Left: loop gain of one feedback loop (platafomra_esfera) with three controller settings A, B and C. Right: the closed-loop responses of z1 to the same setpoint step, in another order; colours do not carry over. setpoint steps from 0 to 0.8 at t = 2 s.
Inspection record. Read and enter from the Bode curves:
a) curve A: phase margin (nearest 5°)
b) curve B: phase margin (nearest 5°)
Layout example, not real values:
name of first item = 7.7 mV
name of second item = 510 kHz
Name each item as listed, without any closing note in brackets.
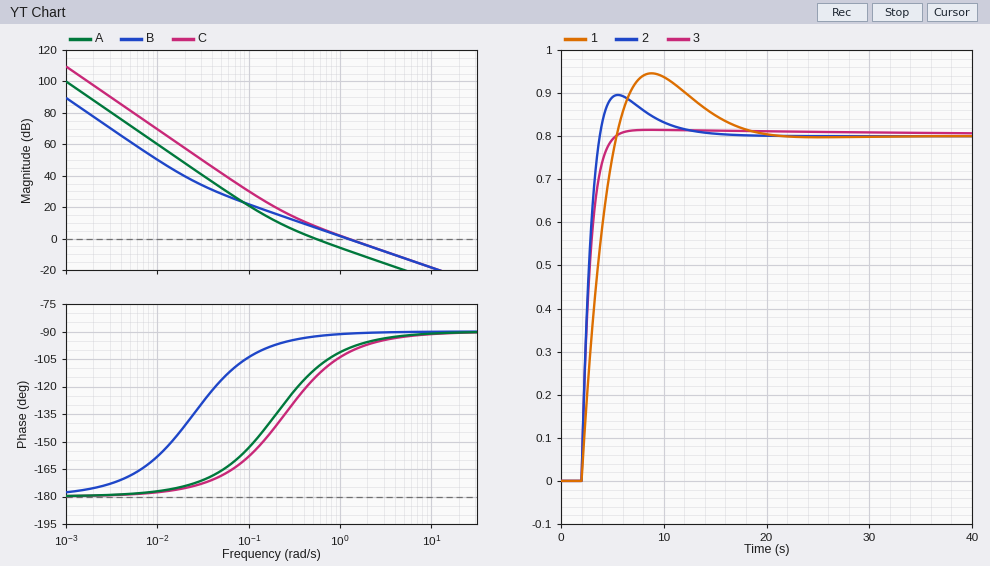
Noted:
curve A: phase margin = 70°
curve B: phase margin = 90°
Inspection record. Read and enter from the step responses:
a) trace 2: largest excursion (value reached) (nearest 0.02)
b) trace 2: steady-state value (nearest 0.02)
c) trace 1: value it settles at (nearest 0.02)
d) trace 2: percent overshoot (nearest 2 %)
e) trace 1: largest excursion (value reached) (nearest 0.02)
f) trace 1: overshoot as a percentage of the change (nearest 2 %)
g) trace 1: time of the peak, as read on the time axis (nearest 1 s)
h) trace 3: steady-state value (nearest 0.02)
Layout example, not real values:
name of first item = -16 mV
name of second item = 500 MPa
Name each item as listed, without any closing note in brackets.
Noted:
trace 2: largest excursion (value reached) = 0.90
trace 2: steady-state value = 0.80
trace 1: value it settles at = 0.80
trace 2: percent overshoot = 12 %
trace 1: largest excursion (value reached) = 0.94
trace 1: overshoot as a percentage of the change = 18 %
trace 1: time of the peak, as read on the time axis = 9 s
trace 3: steady-state value = 0.80
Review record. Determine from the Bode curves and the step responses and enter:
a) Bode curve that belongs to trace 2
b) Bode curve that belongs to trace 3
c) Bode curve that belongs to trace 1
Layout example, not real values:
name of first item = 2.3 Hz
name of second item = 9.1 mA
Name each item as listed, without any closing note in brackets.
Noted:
Bode curve that belongs to trace 2 = C
Bode curve that belongs to trace 3 = B
Bode curve that belongs to trace 1 = A
